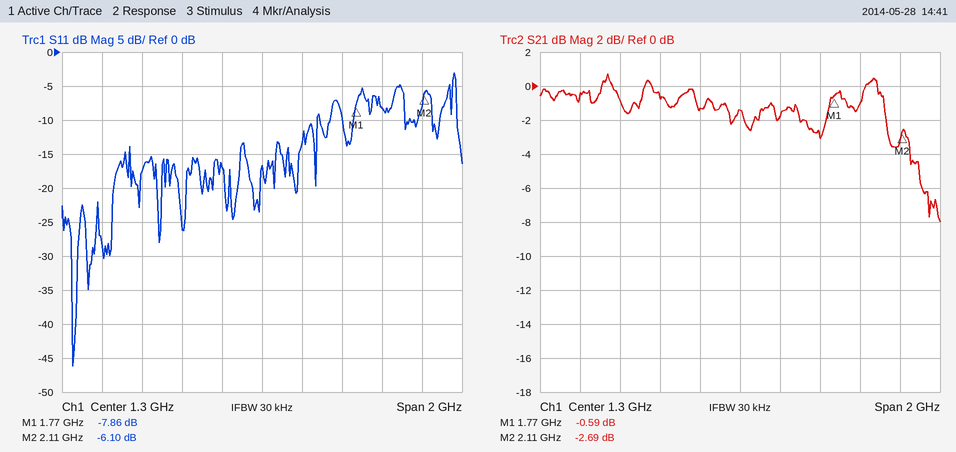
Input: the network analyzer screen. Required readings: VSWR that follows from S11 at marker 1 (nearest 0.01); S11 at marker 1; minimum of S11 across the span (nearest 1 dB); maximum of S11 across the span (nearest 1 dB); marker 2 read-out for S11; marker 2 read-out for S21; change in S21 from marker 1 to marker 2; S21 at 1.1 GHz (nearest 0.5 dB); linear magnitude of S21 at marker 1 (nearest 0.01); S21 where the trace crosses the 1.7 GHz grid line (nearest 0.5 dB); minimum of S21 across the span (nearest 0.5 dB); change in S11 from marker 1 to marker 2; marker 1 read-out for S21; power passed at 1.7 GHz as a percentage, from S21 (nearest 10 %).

2.36
-7.86 dB
-46 dB
-3 dB
-6.10 dB
-2.69 dB
-2.10 dB
-1.5 dB
0.93
-3.0 dB
-8.0 dB
1.76 dB
-0.59 dB
50 %
